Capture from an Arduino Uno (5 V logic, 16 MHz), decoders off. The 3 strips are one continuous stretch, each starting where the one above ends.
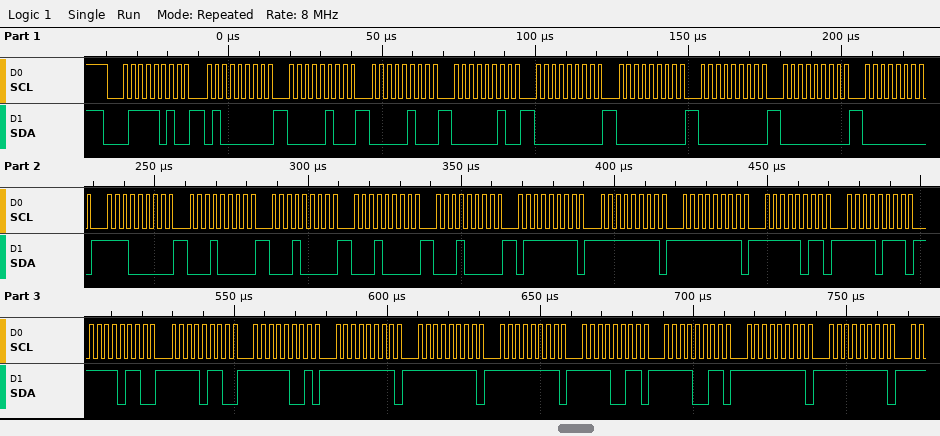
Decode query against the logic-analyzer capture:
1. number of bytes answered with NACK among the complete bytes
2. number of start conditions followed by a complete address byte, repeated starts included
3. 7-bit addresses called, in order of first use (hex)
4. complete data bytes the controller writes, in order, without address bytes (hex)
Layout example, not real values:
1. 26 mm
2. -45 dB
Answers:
1. 0
2. 1
3. 0x3D
4. 40 04 04 02 00 00 00 00 00 E0 10 10 10 10 7F FF FF FB F7 F6 F6 F9 FF FF FF F3 F3 FF FF
